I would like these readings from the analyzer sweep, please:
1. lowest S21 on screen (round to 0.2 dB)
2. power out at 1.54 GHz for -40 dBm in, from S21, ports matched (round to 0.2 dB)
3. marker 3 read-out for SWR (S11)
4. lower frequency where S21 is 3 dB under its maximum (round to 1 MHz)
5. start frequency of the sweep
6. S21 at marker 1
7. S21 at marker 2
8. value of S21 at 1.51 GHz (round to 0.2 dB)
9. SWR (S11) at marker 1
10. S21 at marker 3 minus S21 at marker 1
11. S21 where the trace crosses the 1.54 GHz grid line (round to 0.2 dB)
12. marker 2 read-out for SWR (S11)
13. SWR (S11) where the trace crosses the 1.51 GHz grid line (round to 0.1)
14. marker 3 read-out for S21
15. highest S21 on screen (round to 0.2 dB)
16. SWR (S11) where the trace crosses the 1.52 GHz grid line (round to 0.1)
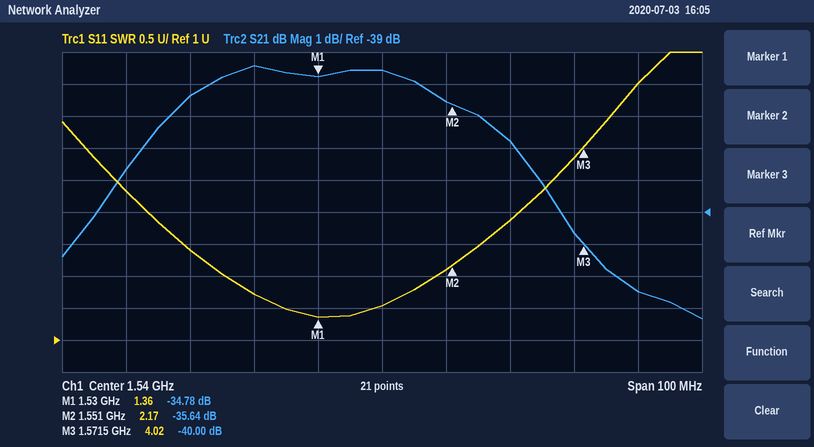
-42.4 dB
-74.6 dBm
4.02
1.501 GHz
1.49 GHz
-34.78 dB
-35.64 dB
-35.4 dB
1.36
-5.22 dB
-34.6 dB
2.17
2.4
-40.00 dB
-34.4 dB
1.7
